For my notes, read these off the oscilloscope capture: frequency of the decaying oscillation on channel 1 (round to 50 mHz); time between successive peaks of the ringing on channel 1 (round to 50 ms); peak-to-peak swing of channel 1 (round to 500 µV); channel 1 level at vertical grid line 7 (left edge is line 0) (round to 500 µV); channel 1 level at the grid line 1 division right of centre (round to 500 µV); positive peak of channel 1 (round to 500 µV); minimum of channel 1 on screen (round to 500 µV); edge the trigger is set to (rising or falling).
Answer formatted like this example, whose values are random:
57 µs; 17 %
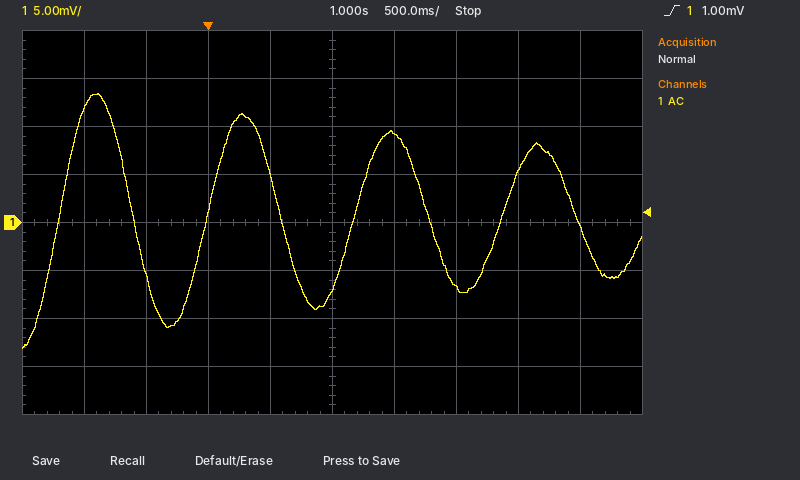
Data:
850 mHz; 1.20 s; 26.5 mV; -7.0 mV; 9.5 mV; 13.5 mV; -13.0 mV; rising
